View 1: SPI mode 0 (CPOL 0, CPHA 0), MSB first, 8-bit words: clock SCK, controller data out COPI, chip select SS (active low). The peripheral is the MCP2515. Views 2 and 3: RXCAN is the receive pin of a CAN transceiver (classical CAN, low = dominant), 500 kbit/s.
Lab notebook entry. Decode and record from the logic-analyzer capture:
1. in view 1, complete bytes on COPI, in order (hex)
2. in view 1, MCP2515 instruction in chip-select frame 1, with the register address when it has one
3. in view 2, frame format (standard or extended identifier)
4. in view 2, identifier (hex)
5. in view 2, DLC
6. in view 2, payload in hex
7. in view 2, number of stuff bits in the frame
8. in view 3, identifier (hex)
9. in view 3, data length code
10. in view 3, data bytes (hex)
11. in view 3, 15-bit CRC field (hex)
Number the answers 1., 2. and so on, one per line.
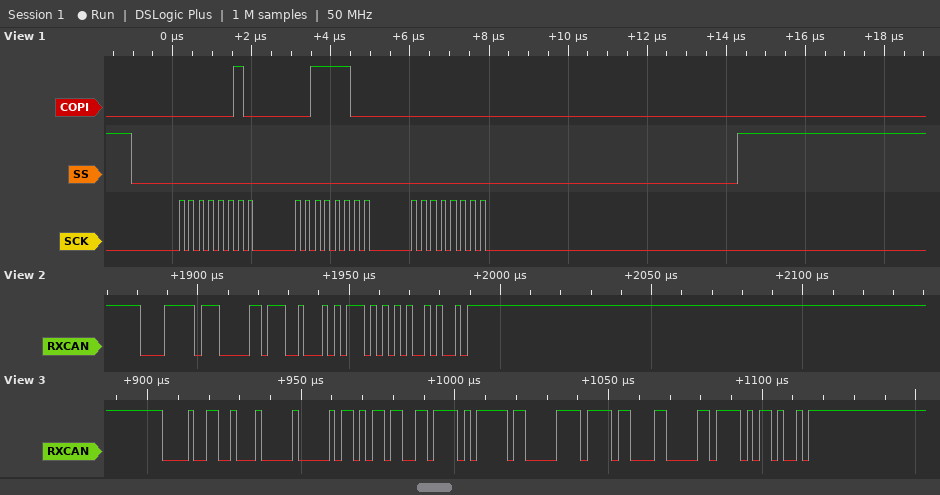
1. 02 3C 00
2. WRITE 0x3C
3. standard
4. 0x0FF
5. 2
6. E4 57
7. 2
8. 0x099
9. 8
10. 00 D6 CD EB F8 3B D8 60
11. 0x5EB4
